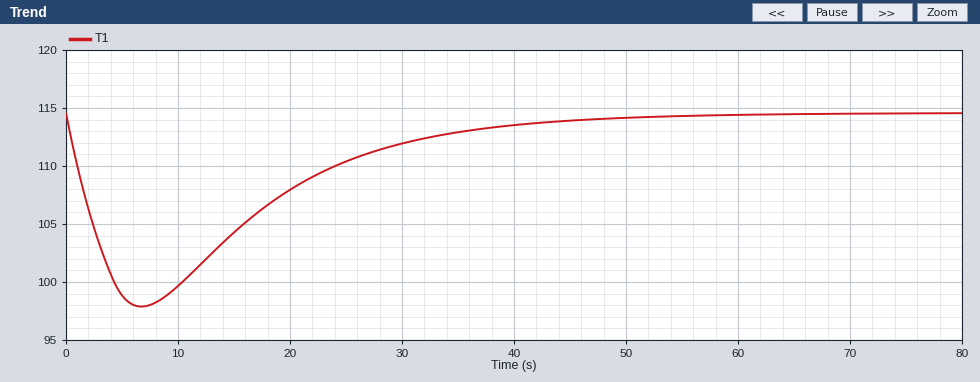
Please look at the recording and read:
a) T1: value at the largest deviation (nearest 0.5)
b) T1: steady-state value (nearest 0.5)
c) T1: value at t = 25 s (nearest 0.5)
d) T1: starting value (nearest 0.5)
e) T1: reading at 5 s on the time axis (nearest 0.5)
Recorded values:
98.0
114.5
110.5
114.5
99.0
